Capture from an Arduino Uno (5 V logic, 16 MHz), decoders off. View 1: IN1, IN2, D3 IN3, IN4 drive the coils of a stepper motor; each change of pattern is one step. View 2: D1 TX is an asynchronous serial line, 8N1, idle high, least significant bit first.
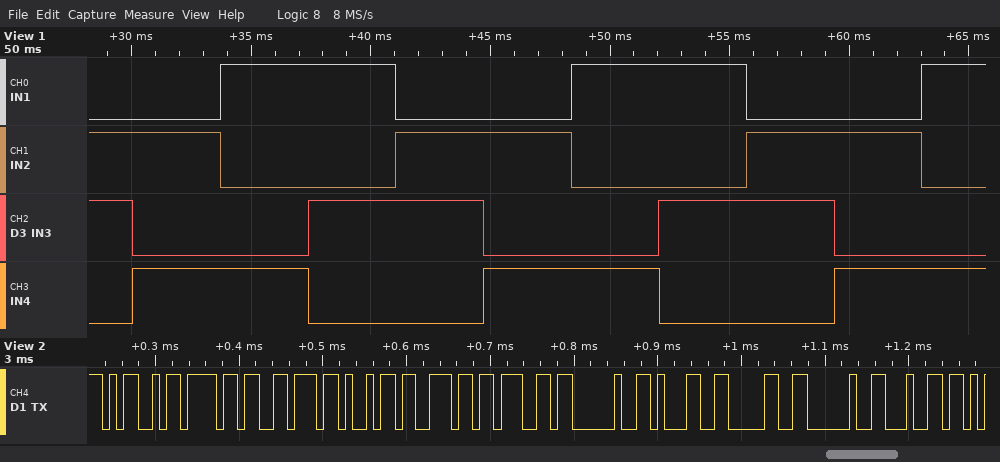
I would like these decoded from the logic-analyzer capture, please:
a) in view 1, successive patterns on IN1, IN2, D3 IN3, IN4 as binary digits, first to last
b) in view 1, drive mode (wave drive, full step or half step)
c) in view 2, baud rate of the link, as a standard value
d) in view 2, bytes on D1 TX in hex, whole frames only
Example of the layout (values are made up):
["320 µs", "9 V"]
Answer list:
["0110 0101 1001 1010 0110 0101 1001 1010 0110 0101 1001", "full step", "115200 baud", "0x4D 0x6F 0x76 0x69 0x6E 0x67 0x20 0x31 0x30 0x20 0x64"]
